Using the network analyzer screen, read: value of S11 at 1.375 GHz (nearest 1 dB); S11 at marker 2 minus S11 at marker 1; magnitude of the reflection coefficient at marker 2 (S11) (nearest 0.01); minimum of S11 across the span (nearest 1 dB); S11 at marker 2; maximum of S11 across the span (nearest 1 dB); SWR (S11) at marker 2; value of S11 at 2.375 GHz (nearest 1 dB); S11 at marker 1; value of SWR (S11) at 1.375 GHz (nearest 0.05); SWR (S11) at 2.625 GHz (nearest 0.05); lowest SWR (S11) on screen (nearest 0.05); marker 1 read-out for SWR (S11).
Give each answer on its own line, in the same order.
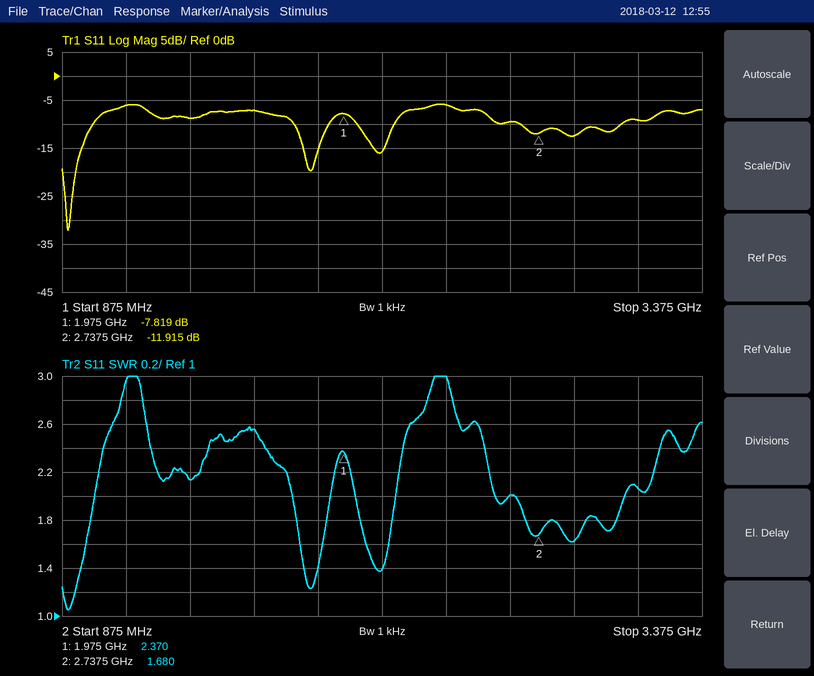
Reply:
-9 dB
-4.096 dB
0.25
-32 dB
-11.915 dB
-6 dB
1.680
-6 dB
-7.819 dB
2.15
2.00
1.05
2.370
